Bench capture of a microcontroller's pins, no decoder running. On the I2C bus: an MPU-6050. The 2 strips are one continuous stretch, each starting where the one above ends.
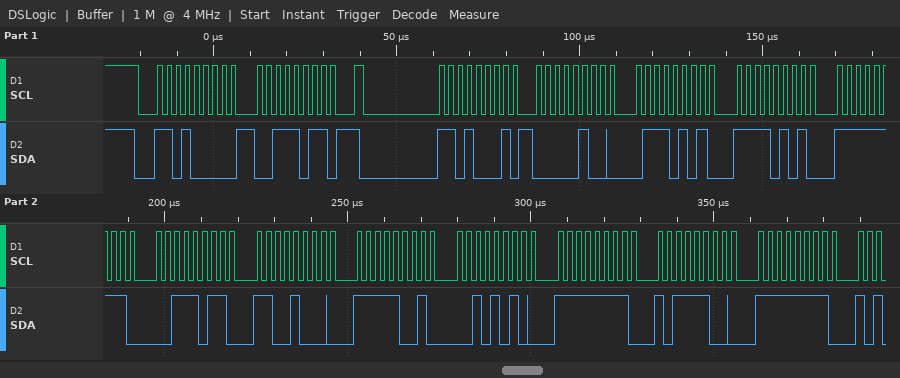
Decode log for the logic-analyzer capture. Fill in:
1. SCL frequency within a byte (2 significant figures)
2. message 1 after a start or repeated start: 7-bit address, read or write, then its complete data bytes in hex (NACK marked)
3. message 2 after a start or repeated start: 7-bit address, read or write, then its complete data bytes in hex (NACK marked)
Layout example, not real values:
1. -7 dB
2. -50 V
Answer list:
1. 400 kHz
2. 0x68 write: 3B
3. 0x68 read: 04 75 F5 FF 3B C8 F9 2A FF BC FF
